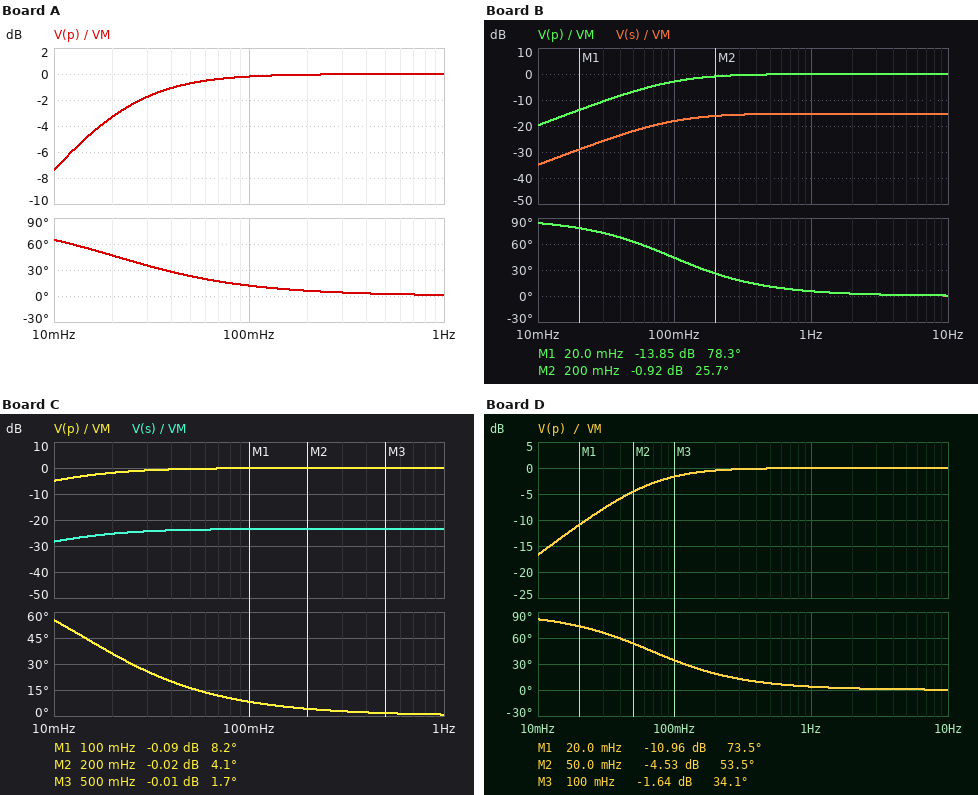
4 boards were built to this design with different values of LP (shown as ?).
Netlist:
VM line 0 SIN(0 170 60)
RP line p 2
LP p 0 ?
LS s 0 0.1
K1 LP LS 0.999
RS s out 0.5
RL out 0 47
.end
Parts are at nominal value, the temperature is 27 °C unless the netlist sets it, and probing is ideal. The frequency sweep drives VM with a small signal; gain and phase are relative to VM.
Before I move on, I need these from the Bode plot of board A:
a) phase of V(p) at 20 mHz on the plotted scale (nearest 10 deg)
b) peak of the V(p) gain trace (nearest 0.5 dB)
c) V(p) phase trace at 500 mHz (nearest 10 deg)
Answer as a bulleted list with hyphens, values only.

- 50 deg
- 0 dB
- 0 deg
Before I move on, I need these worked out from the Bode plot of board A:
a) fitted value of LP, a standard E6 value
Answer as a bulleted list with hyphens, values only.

- 15 H
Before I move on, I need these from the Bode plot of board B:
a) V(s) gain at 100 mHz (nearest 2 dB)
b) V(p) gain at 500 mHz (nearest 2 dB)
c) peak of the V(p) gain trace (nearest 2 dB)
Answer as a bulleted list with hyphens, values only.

- -18 dB
- 0 dB
- 0 dB
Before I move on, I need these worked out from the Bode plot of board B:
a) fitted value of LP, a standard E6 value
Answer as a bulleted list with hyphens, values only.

- 3.3 H
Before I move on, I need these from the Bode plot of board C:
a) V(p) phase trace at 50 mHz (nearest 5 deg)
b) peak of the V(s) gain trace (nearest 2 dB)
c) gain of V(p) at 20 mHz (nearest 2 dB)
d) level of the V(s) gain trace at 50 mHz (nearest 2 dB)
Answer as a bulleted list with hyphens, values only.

- 15 deg
- -24 dB
- -2 dB
- -24 dB
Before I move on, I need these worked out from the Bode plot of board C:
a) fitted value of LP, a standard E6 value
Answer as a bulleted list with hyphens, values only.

- 22 H
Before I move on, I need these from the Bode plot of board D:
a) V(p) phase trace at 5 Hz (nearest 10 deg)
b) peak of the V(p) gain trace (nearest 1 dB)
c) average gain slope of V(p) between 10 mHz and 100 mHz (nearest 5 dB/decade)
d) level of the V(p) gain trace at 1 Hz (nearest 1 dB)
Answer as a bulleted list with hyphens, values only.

- 0 deg
- 0 dB
- 15 dB/decade
- 0 dB
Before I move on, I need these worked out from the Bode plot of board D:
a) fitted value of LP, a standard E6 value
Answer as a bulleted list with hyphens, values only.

- 4.7 H
